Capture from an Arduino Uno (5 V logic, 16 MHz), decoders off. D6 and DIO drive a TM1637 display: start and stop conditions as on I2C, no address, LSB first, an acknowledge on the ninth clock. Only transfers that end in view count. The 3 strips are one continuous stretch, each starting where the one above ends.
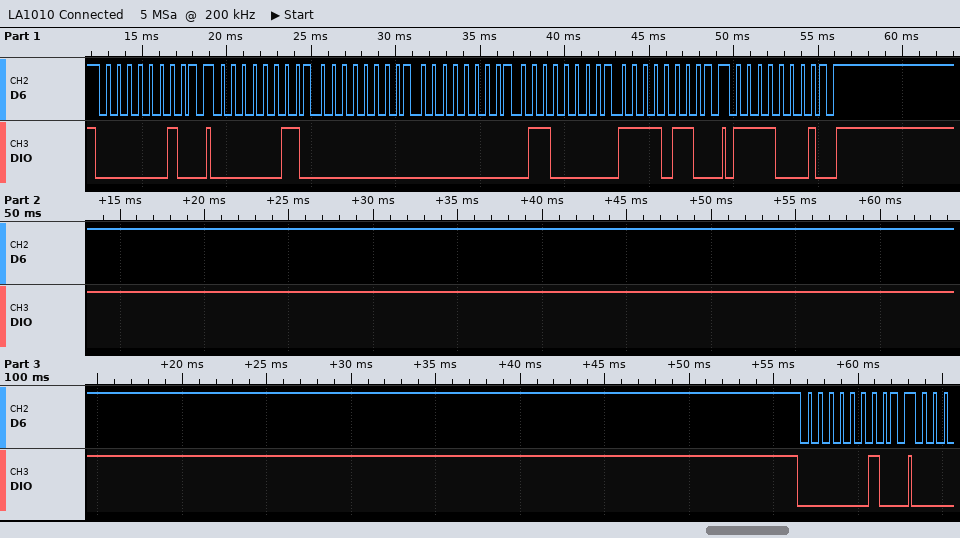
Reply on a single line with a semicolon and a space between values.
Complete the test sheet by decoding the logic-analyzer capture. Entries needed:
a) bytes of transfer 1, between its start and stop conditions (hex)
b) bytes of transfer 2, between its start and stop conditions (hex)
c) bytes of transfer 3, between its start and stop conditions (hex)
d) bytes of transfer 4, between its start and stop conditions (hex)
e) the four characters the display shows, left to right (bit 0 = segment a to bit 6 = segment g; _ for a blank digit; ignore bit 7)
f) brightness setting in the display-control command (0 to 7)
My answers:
40; C0 00 00 06 6F; 8F; 40; __19; 7
